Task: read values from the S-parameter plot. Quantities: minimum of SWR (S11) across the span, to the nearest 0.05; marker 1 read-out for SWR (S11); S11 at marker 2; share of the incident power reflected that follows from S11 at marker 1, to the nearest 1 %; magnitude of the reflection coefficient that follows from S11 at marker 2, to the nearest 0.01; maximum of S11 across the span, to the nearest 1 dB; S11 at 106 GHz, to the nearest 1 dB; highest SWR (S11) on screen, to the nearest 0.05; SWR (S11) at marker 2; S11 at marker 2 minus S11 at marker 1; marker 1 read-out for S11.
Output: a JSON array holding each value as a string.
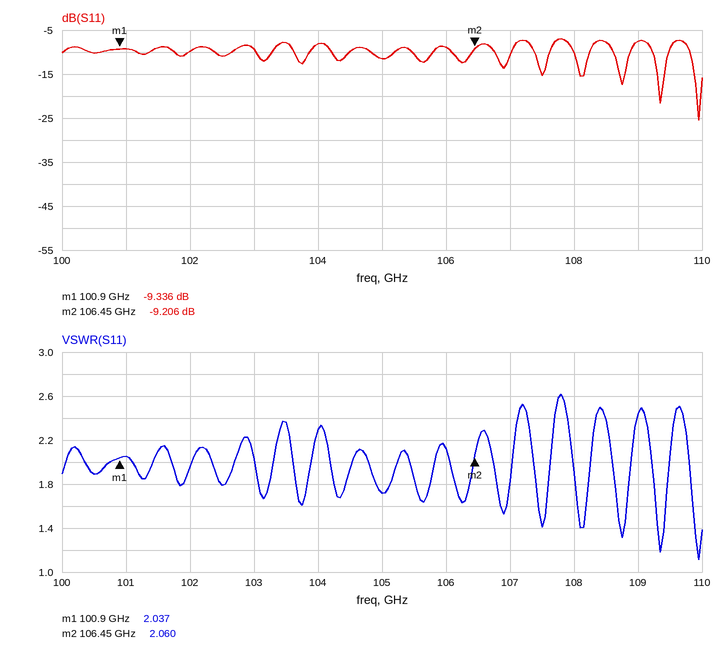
["1.10", "2.037", "-9.206 dB", "12 %", "0.35", "-7 dB", "-9 dB", "2.60", "2.060", "0.130 dB", "-9.336 dB"]
